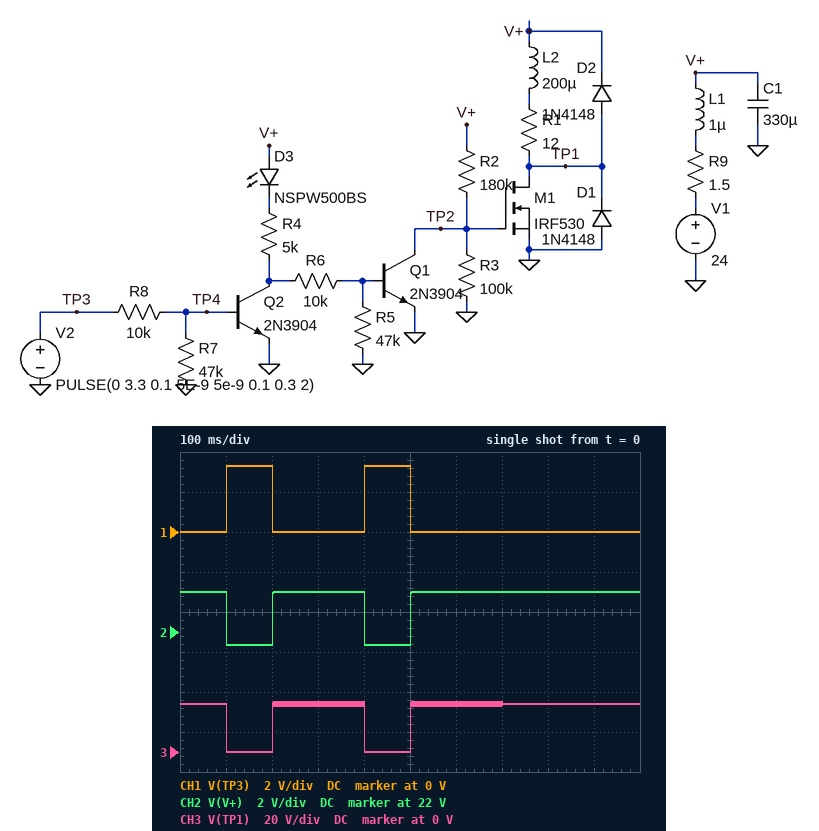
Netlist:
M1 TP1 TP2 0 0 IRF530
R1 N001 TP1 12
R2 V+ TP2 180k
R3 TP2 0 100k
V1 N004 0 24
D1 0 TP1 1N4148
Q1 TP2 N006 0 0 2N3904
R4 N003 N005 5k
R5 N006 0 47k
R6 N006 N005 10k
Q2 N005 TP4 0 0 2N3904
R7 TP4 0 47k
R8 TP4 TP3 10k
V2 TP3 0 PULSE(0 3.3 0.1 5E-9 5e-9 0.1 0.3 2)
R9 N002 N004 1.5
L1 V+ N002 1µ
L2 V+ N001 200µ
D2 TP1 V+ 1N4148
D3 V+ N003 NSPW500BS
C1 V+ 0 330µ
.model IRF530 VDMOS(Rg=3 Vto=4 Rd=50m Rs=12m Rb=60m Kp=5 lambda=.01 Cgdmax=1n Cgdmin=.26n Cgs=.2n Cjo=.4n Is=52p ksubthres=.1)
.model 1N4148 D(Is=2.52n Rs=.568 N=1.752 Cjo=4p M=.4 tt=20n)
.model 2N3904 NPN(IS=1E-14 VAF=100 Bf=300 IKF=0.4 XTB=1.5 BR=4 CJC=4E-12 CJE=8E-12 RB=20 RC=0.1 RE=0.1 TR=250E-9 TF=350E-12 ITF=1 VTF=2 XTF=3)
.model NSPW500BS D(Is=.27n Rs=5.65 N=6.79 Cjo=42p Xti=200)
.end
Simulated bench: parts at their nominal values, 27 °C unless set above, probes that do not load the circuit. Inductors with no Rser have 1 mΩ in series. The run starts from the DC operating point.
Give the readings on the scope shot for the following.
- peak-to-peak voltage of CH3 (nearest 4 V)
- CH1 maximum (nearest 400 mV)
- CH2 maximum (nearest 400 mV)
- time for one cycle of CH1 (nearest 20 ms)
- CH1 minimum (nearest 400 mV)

24 V
3.2 V
24.0 V
300 ms
0 V
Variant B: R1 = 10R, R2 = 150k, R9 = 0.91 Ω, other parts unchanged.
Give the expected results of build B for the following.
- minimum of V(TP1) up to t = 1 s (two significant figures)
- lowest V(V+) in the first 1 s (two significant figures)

230 mV
22 V
